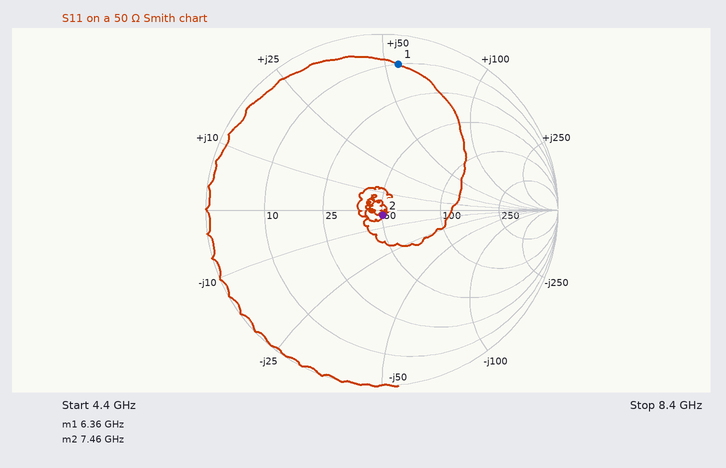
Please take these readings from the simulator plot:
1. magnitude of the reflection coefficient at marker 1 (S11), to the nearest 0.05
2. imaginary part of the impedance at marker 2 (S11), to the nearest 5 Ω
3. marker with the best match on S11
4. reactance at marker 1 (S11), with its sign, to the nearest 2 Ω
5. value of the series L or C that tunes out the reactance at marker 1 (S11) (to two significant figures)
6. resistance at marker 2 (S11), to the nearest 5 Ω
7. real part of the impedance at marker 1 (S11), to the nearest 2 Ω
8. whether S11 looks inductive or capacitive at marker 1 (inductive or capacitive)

0.85
-5 Ω
marker 2
+54 Ω
460 fF
50 Ω
10 Ω
inductive
